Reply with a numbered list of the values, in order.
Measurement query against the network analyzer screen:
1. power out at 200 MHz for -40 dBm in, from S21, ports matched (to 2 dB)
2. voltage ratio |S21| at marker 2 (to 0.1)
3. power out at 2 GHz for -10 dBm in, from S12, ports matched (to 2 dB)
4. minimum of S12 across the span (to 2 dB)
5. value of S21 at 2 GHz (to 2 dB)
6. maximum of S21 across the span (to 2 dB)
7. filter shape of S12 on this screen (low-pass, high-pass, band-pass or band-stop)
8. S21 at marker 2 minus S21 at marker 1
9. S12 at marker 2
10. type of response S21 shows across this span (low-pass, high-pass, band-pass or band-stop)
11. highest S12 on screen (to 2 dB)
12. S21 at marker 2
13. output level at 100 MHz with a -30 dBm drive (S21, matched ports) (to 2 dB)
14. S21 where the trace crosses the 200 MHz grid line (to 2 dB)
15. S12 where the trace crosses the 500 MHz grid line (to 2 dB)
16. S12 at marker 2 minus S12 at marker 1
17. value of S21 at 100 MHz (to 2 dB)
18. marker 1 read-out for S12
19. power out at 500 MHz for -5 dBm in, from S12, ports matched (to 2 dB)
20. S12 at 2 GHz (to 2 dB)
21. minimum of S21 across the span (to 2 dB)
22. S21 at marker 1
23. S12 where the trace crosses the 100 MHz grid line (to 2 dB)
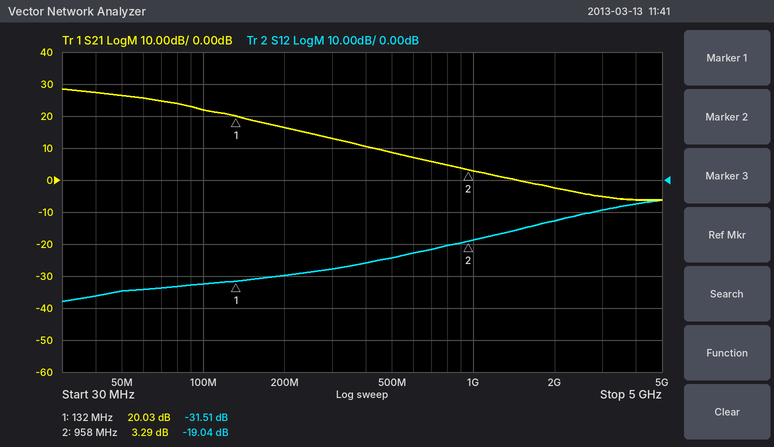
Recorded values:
1. -24 dBm
2. 1.5
3. -22 dBm
4. -38 dB
5. -2 dB
6. 28 dB
7. high-pass
8. -16.74 dB
9. -19.04 dB
10. low-pass
11. -6 dB
12. 3.29 dB
13. -8 dBm
14. 16 dB
15. -24 dB
16. 12.47 dB
17. 22 dB
18. -31.51 dB
19. -30 dBm
20. -12 dB
21. -6 dB
22. 20.03 dB
23. -32 dB
